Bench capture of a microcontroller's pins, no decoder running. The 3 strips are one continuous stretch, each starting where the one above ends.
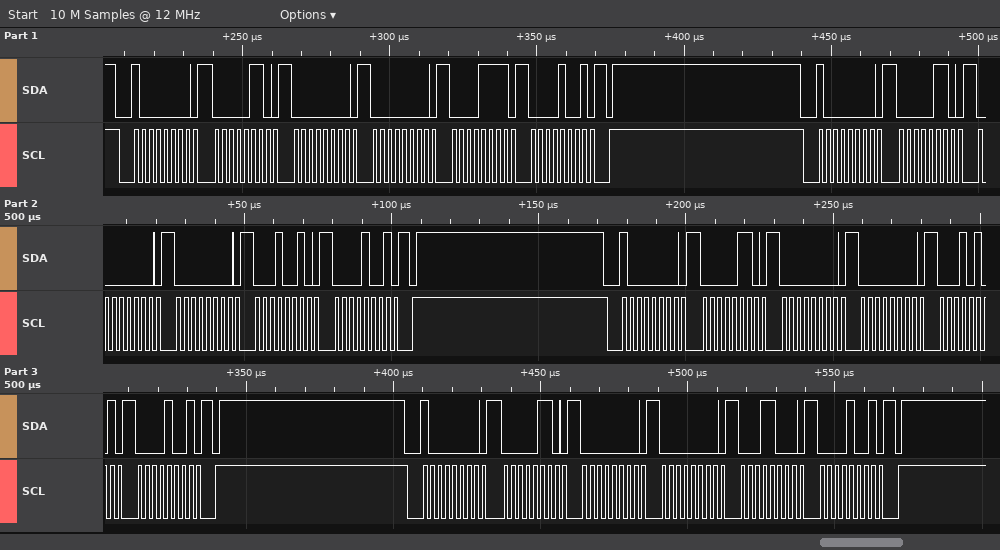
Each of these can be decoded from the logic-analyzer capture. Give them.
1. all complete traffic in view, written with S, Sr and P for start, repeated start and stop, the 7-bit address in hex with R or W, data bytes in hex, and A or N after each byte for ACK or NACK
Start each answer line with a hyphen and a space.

- S 40W A 06 A 00 A 00 A 0F A 09 A P S 40W A 06 A 00 A 00 A 12 A 09 A P S 40W A 06 A 00 A 00 A 15 A 09 A P S 40W A 06 A 00 A 00 A 18 A 09 A P
